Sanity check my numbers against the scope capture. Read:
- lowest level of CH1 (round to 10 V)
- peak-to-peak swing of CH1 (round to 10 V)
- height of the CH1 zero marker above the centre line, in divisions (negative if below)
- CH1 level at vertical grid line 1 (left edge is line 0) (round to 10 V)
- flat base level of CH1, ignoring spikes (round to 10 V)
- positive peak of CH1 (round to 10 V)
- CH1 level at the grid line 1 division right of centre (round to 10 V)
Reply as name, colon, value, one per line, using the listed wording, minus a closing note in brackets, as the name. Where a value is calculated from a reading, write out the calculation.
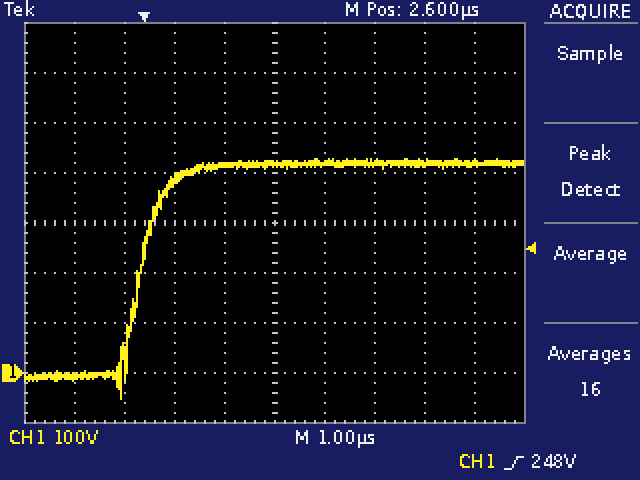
lowest level of CH1: -50 V
peak-to-peak swing of CH1: 430 V − (-50 V) = 480 V
height of the CH1 zero marker above the centre line, in divisions: -3.0 div
CH1 level at vertical grid line 1 (left edge is line 0): -10 V
flat base level of CH1, ignoring spikes: -10 V
positive peak of CH1: 430 V
CH1 level at the grid line 1 division right of centre: 420 V
